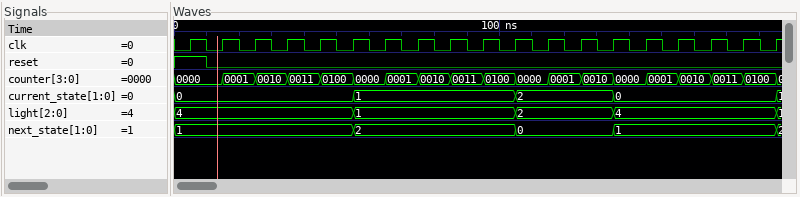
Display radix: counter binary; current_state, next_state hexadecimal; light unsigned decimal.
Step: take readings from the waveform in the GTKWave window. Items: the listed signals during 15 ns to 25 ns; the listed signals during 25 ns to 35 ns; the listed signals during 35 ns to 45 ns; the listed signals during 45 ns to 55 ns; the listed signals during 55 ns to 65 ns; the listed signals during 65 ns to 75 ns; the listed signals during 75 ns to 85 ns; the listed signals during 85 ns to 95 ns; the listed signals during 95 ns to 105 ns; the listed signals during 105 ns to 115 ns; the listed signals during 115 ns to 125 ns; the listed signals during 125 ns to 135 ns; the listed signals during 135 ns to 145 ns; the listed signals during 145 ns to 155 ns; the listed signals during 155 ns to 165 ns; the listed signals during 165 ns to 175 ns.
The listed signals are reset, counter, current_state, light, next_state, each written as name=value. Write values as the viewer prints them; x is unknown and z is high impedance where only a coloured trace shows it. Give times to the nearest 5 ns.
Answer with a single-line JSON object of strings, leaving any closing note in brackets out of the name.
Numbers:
{"the listed signals during 15 ns to 25 ns": "reset=0, counter=0001, current_state=0, light=4, next_state=1", "the listed signals during 25 ns to 35 ns": "reset=0, counter=0010, current_state=0, light=4, next_state=1", "the listed signals during 35 ns to 45 ns": "reset=0, counter=0011, current_state=0, light=4, next_state=1", "the listed signals during 45 ns to 55 ns": "reset=0, counter=0100, current_state=0, light=4, next_state=1", "the listed signals during 55 ns to 65 ns": "reset=0, counter=0000, current_state=1, light=1, next_state=2", "the listed signals during 65 ns to 75 ns": "reset=0, counter=0001, current_state=1, light=1, next_state=2", "the listed signals during 75 ns to 85 ns": "reset=0, counter=0010, current_state=1, light=1, next_state=2", "the listed signals during 85 ns to 95 ns": "reset=0, counter=0011, current_state=1, light=1, next_state=2", "the listed signals during 95 ns to 105 ns": "reset=0, counter=0100, current_state=1, light=1, next_state=2", "the listed signals during 105 ns to 115 ns": "reset=0, counter=0000, current_state=2, light=2, next_state=0", "the listed signals during 115 ns to 125 ns": "reset=0, counter=0001, current_state=2, light=2, next_state=0", "the listed signals during 125 ns to 135 ns": "reset=0, counter=0010, current_state=2, light=2, next_state=0", "the listed signals during 135 ns to 145 ns": "reset=0, counter=0000, current_state=0, light=4, next_state=1", "the listed signals during 145 ns to 155 ns": "reset=0, counter=0001, current_state=0, light=4, next_state=1", "the listed signals during 155 ns to 165 ns": "reset=0, counter=0010, current_state=0, light=4, next_state=1", "the listed signals during 165 ns to 175 ns": "reset=0, counter=0011, current_state=0, light=4, next_state=1"}
